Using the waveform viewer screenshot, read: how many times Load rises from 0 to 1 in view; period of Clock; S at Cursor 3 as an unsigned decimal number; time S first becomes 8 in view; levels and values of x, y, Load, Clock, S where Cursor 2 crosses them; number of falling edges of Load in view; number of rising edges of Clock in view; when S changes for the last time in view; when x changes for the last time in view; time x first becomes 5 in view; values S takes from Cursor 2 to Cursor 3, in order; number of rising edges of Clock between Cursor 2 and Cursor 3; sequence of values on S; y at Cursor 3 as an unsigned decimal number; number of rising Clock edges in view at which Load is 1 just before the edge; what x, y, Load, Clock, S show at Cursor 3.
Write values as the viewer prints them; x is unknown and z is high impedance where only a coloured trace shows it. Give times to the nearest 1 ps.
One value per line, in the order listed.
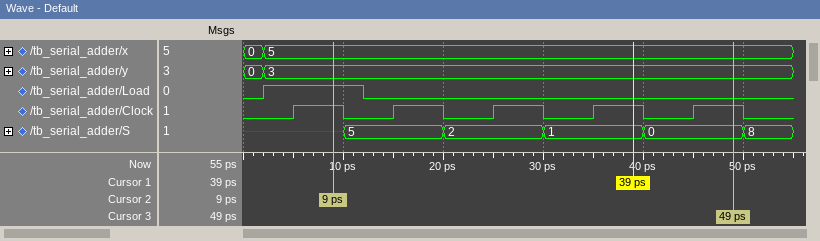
1
10 ps
0
50 ps
x=5, y=3, Load=1, Clock=1, S=x
1
5
50 ps
2 ps
2 ps
x, 5, 2, 1, 0
4
x, 5, 2, 1, 0, 8
3
1
x=5, y=3, Load=0, Clock=1, S=0
